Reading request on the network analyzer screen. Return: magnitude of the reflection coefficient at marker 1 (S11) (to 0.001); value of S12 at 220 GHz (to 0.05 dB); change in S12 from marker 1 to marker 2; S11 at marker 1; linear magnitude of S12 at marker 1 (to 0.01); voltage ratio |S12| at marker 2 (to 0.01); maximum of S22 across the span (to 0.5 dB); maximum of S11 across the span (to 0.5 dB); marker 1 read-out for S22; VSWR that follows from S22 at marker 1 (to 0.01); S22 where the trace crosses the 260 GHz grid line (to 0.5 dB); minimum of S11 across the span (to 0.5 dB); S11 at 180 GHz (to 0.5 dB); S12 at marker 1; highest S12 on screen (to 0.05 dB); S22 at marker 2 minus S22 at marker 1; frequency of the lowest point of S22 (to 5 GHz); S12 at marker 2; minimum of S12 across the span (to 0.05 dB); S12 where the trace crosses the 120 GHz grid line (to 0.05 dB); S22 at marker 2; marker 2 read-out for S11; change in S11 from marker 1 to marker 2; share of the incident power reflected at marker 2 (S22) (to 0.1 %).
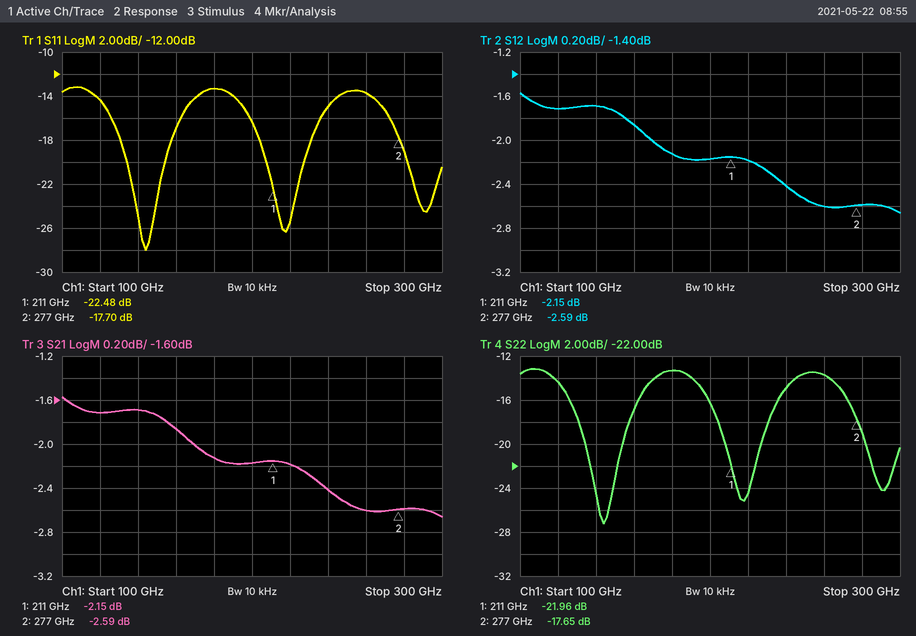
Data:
0.075
-2.20 dB
-0.44 dB
-22.48 dB
0.78
0.74
-13.0 dB
-13.0 dB
-21.96 dB
1.17
-13.5 dB
-28.0 dB
-13.5 dB
-2.15 dB
-1.55 dB
4.31 dB
145 GHz
-2.59 dB
-2.65 dB
-1.70 dB
-17.65 dB
-17.70 dB
4.78 dB
1.7 %
